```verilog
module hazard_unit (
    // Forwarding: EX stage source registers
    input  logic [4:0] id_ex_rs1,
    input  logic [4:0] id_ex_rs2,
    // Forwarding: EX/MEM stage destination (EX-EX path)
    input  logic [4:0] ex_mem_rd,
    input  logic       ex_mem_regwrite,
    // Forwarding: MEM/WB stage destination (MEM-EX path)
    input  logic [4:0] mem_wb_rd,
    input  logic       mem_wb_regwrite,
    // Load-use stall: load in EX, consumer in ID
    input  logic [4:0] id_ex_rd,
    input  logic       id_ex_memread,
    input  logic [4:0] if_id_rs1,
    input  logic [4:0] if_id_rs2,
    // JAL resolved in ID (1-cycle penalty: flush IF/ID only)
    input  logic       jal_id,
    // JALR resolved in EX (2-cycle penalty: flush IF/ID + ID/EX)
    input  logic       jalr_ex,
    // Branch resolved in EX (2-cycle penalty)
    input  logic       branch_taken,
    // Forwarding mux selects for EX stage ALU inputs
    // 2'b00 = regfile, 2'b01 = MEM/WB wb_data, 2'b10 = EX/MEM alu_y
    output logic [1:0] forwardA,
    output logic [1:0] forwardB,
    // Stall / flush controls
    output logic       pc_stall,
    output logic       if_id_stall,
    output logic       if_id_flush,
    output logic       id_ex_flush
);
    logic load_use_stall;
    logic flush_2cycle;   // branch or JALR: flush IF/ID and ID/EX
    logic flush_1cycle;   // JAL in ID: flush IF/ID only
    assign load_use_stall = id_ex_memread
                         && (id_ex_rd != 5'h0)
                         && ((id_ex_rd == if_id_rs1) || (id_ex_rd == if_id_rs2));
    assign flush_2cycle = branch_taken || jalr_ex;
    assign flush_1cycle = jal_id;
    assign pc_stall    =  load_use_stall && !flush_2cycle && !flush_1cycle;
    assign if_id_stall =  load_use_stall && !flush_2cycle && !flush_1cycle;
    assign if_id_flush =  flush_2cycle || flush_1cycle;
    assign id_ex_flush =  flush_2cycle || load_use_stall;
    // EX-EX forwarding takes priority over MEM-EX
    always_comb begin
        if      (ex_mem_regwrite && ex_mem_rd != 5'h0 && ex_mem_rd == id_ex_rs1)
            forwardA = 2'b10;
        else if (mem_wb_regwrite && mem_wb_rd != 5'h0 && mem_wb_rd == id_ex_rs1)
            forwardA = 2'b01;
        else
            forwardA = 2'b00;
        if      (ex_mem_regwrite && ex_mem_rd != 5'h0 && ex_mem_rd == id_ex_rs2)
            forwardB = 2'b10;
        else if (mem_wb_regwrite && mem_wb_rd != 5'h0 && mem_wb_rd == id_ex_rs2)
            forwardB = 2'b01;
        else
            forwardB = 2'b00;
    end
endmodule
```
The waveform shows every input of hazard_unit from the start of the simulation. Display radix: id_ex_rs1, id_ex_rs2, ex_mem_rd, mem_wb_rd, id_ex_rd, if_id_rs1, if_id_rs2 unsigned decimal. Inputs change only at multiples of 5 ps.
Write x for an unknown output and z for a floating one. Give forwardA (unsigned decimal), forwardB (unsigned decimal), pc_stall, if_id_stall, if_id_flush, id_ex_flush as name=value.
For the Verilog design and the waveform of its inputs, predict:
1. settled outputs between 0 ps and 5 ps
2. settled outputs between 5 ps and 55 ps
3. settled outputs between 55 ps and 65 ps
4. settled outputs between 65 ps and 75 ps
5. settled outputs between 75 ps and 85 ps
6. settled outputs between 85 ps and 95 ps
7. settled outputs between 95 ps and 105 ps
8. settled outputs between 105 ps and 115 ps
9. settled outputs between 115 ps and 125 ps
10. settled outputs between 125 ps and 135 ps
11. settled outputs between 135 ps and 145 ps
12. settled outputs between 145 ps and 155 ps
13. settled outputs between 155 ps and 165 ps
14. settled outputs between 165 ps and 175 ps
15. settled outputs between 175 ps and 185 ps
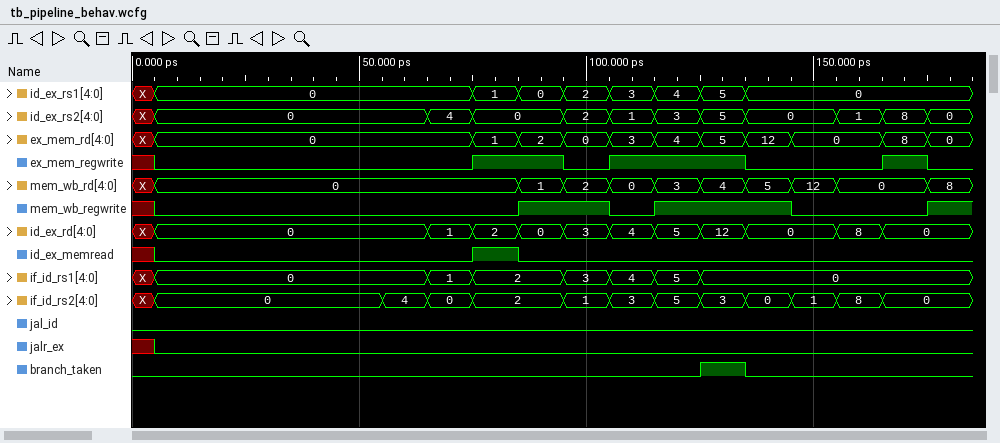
forwardA=0, forwardB=0, pc_stall=x, if_id_stall=x, if_id_flush=x, id_ex_flush=x
forwardA=0, forwardB=0, pc_stall=0, if_id_stall=0, if_id_flush=0, id_ex_flush=0
forwardA=0, forwardB=0, pc_stall=0, if_id_stall=0, if_id_flush=0, id_ex_flush=0
forwardA=0, forwardB=0, pc_stall=0, if_id_stall=0, if_id_flush=0, id_ex_flush=0
forwardA=2, forwardB=0, pc_stall=1, if_id_stall=1, if_id_flush=0, id_ex_flush=1
forwardA=0, forwardB=0, pc_stall=0, if_id_stall=0, if_id_flush=0, id_ex_flush=0
forwardA=1, forwardB=1, pc_stall=0, if_id_stall=0, if_id_flush=0, id_ex_flush=0
forwardA=2, forwardB=0, pc_stall=0, if_id_stall=0, if_id_flush=0, id_ex_flush=0
forwardA=2, forwardB=1, pc_stall=0, if_id_stall=0, if_id_flush=0, id_ex_flush=0
forwardA=2, forwardB=2, pc_stall=0, if_id_stall=0, if_id_flush=1, id_ex_flush=1
forwardA=0, forwardB=0, pc_stall=0, if_id_stall=0, if_id_flush=0, id_ex_flush=0
forwardA=0, forwardB=0, pc_stall=0, if_id_stall=0, if_id_flush=0, id_ex_flush=0
forwardA=0, forwardB=0, pc_stall=0, if_id_stall=0, if_id_flush=0, id_ex_flush=0
forwardA=0, forwardB=2, pc_stall=0, if_id_stall=0, if_id_flush=0, id_ex_flush=0
forwardA=0, forwardB=0, pc_stall=0, if_id_stall=0, if_id_flush=0, id_ex_flush=0
